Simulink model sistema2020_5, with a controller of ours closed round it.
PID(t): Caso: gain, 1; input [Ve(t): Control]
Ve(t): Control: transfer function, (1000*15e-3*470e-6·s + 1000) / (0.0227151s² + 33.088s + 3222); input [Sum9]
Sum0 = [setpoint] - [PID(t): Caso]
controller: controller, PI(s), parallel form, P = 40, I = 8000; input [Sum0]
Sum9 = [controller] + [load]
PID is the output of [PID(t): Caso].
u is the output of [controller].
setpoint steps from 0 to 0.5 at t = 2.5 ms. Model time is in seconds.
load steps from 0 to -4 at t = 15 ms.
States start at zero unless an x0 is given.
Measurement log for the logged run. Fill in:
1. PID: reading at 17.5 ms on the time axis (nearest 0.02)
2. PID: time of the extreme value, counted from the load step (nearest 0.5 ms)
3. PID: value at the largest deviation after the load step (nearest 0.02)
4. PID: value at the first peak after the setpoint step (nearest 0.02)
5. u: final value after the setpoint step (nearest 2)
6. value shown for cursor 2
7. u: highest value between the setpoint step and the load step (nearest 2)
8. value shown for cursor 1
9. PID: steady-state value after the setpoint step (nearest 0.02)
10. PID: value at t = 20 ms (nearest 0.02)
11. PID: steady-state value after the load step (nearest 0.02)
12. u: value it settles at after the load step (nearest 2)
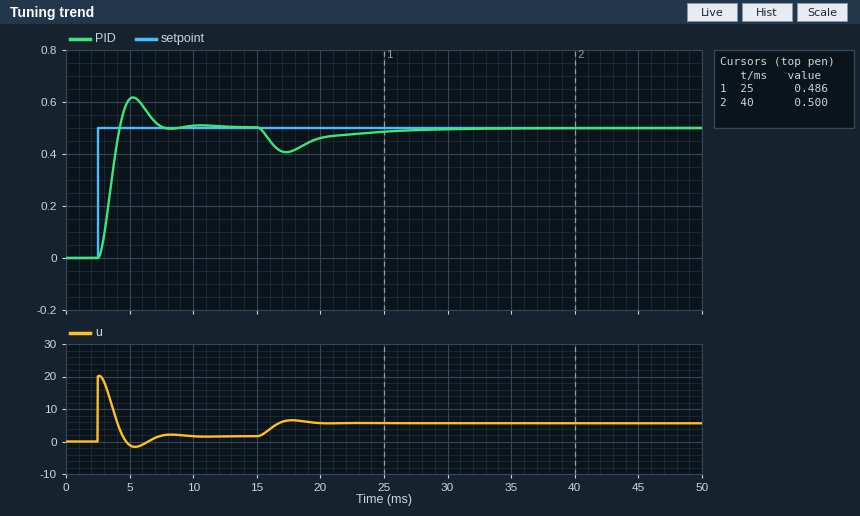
0.40
2.5 ms
0.40
0.62
2
0.500
20
0.486
0.50
0.46
0.50
6
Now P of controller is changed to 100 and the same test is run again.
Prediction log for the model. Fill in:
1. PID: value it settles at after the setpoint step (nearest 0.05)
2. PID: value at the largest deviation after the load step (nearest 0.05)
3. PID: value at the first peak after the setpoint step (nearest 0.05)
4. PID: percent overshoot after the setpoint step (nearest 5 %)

0.50
0.45
0.65
30 %
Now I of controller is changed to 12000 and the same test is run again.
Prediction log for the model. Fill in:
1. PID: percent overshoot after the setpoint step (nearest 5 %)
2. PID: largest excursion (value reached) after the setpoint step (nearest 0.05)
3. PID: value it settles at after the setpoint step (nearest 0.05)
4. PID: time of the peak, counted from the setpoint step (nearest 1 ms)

30 %
0.65
0.50
3 ms
